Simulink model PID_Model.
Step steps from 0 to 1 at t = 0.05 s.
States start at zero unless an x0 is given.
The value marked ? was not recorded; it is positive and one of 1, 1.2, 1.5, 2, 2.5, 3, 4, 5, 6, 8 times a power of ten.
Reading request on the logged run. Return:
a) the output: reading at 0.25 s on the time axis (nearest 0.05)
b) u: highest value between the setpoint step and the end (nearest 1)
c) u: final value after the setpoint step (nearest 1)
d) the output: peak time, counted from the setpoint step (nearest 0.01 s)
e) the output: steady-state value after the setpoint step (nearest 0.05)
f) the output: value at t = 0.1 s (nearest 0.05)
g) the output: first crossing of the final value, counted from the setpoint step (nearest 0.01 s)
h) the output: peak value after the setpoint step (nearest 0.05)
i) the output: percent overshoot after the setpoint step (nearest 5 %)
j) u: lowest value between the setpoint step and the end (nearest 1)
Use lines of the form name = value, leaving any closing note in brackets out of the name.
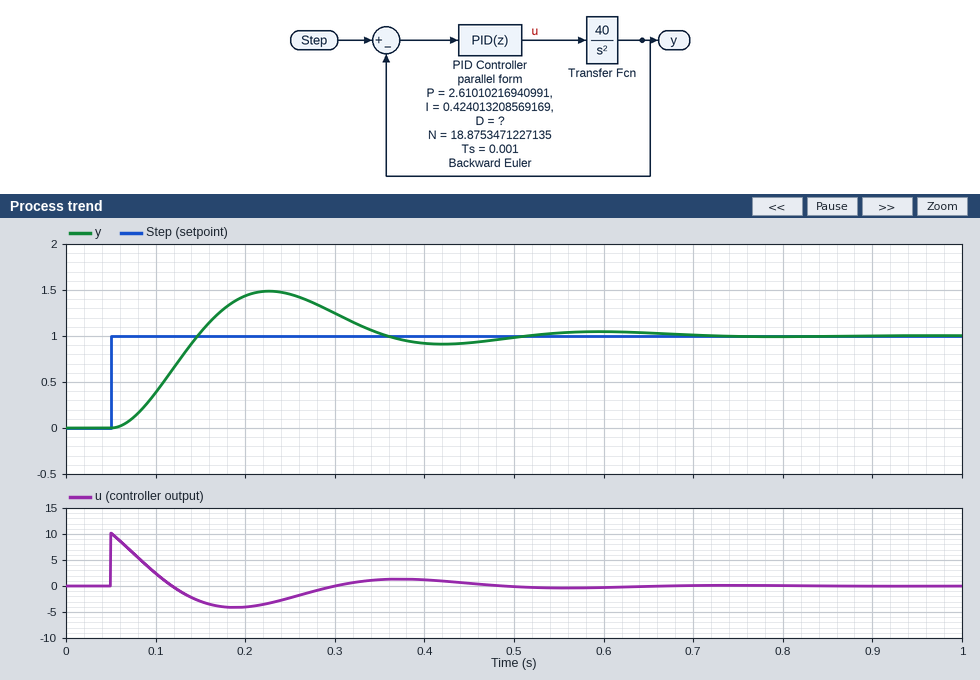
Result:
the output: reading at 0.25 s on the time axis = 1.45
u: highest value between the setpoint step and the end = 10
u: final value after the setpoint step = 0
the output: peak time, counted from the setpoint step = 0.18 s
the output: steady-state value after the setpoint step = 1.00
the output: value at t = 0.1 s = 0.40
the output: first crossing of the final value, counted from the setpoint step = 0.10 s
the output: peak value after the setpoint step = 1.50
the output: percent overshoot after the setpoint step = 50 %
u: lowest value between the setpoint step and the end = -4
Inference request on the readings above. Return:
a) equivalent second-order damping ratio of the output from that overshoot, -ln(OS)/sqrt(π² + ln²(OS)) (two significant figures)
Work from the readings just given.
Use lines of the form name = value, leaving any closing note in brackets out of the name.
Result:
equivalent second-order damping ratio of the output from that overshoot, -ln(OS)/sqrt(π² + ln²(OS)) = 0.22
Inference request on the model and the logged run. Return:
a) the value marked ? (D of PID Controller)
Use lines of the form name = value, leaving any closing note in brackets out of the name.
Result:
the value marked ? = 0.4
